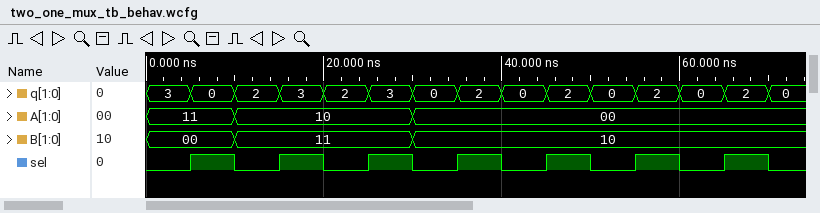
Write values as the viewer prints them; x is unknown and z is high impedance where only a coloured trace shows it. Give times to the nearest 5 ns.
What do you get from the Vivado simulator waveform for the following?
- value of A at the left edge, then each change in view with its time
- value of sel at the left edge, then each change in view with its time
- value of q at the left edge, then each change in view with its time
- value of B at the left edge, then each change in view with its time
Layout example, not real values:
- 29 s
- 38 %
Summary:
- 11, 10 at 10 ns, 00 at 30 ns
- 0, 1 at 5 ns, 0 at 10 ns, 1 at 15 ns, 0 at 20 ns, 1 at 25 ns, 0 at 30 ns, 1 at 35 ns, 0 at 40 ns, 1 at 45 ns, 0 at 50 ns, 1 at 55 ns, 0 at 60 ns, 1 at 65 ns, 0 at 70 ns
- 3, 0 at 5 ns, 2 at 10 ns, 3 at 15 ns, 2 at 20 ns, 3 at 25 ns, 0 at 30 ns, 2 at 35 ns, 0 at 40 ns, 2 at 45 ns, 0 at 50 ns, 2 at 55 ns, 0 at 60 ns, 2 at 65 ns, 0 at 70 ns
- 00, 11 at 10 ns, 10 at 30 ns
